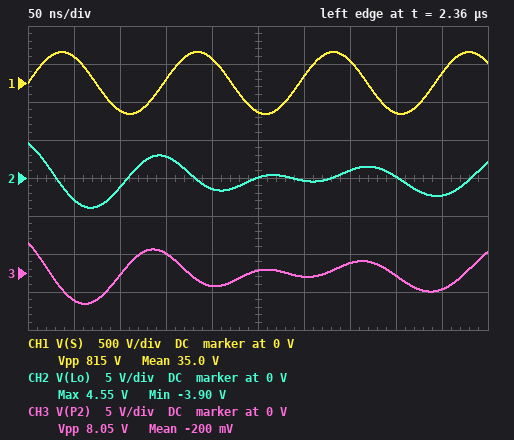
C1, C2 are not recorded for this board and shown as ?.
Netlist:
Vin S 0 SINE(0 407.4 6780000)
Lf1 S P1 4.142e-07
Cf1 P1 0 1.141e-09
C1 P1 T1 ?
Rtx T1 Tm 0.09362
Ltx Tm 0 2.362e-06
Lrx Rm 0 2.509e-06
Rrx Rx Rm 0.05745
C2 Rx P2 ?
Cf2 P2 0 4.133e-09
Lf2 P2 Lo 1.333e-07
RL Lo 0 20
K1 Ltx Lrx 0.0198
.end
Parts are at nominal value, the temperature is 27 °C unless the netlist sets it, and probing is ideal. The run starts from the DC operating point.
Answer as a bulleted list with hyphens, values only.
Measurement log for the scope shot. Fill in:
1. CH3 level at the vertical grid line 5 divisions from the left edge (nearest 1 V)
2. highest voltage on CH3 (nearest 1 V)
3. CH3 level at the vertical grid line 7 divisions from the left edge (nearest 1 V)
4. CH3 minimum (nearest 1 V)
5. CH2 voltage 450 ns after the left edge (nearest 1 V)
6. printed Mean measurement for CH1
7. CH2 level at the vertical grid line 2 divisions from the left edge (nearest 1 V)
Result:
- 0 V
- 4 V
- 1 V
- -4 V
- -2 V
- 35.0 V
- -1 V
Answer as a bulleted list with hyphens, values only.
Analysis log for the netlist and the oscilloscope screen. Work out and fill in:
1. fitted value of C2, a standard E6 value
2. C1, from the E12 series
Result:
- 680 pF
- 150 pF
